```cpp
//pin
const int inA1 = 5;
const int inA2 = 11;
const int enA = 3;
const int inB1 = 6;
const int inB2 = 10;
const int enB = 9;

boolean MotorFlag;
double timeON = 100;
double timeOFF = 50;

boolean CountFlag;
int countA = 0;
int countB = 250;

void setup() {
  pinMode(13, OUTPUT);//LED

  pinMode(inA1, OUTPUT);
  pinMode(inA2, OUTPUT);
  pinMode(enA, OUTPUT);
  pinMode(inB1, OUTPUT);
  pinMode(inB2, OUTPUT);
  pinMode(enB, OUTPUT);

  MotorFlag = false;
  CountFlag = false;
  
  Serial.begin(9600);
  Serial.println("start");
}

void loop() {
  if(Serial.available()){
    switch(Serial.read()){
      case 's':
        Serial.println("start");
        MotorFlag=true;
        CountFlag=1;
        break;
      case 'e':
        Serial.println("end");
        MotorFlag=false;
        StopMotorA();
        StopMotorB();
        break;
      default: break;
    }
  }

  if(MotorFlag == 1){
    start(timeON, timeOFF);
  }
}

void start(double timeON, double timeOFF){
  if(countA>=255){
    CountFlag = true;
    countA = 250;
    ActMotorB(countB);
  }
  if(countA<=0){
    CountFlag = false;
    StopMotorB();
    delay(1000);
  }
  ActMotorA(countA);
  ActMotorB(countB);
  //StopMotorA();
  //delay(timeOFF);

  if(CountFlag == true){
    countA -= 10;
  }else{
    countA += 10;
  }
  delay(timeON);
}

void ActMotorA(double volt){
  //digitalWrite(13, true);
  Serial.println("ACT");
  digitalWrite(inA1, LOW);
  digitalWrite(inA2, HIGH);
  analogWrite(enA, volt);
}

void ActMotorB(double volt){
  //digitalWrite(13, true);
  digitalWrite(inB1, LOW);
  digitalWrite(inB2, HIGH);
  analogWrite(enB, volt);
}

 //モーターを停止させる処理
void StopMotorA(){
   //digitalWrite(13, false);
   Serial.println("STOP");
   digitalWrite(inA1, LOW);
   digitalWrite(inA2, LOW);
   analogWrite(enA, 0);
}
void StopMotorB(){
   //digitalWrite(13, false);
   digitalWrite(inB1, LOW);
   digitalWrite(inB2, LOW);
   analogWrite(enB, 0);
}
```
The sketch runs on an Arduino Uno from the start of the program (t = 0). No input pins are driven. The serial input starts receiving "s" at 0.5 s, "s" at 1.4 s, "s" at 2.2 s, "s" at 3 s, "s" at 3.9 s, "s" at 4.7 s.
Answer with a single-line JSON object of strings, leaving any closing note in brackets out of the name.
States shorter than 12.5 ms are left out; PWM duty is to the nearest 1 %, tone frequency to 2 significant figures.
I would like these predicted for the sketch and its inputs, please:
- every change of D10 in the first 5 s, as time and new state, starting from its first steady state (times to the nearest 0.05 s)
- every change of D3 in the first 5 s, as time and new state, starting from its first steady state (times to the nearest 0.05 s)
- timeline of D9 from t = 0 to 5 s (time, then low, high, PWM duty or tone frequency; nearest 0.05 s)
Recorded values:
{"every change of D10 in the first 5 s, as time and new state, starting from its first steady state": "0 s low; 1.5 s high; 1.7 s low; 2.7 s high; 2.9 s low; 3.9 s high; 4.1 s low", "every change of D3 in the first 5 s, as time and new state, starting from its first steady state": "0 s low; 1.6 s PWM 4 %; 2.7 s low; 2.8 s PWM 4 %; 3.9 s low; 4 s PWM 4 %", "timeline of D9 from t = 0 to 5 s": "0 s low; 1.5 s PWM 98 %; 1.7 s low; 2.7 s PWM 98 %; 2.9 s low; 3.9 s PWM 98 %; 4.1 s low"}
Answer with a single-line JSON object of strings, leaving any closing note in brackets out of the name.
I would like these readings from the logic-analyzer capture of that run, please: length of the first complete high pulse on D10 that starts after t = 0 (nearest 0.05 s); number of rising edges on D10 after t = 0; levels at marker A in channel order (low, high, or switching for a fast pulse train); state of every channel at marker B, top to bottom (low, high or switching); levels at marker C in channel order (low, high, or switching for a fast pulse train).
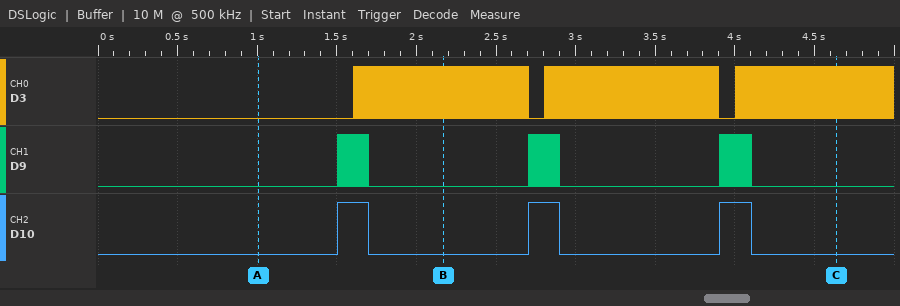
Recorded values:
{"length of the first complete high pulse on D10 that starts after t = 0": "0.20 s", "number of rising edges on D10 after t = 0": "3", "levels at marker A in channel order": "D3 low, D9 low, D10 low", "state of every channel at marker B, top to bottom": "D3 switching, D9 low, D10 low", "levels at marker C in channel order": "D3 switching, D9 low, D10 low"}
